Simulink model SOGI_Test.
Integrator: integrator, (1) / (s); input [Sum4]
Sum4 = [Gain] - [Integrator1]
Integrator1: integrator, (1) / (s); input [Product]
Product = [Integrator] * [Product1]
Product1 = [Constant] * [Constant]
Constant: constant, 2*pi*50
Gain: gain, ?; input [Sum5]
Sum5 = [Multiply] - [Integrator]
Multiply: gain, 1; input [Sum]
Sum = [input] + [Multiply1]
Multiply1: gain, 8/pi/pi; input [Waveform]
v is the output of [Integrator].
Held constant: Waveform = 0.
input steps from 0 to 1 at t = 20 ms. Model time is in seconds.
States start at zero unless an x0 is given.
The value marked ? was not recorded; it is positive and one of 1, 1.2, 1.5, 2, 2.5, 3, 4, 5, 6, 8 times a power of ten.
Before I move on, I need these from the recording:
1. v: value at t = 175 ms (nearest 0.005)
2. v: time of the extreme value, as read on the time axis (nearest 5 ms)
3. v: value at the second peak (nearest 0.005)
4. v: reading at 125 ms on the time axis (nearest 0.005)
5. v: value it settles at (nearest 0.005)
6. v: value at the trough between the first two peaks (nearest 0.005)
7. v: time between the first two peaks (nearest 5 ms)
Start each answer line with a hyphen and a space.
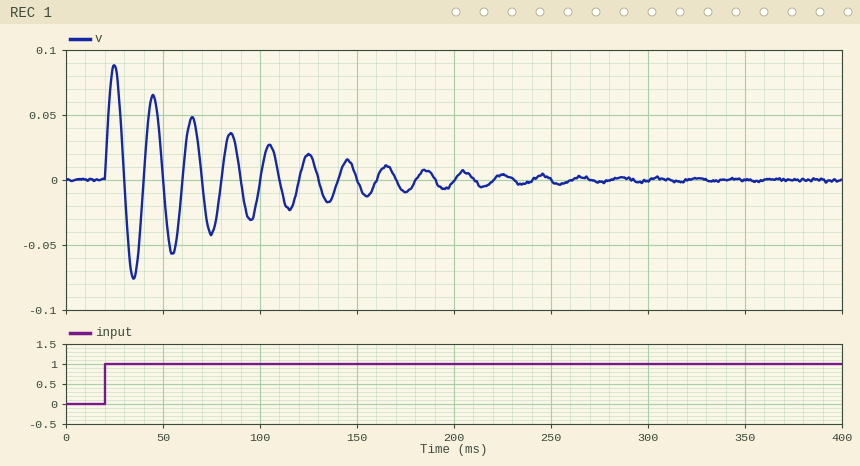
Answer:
- -0.010
- 25 ms
- 0.065
- 0.020
- 0.000
- -0.075
- 20 ms
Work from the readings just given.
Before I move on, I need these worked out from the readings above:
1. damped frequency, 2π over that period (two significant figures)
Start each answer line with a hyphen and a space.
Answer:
- 0.31 rad/ms
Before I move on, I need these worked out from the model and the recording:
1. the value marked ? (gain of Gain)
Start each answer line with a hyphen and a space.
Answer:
- 30
